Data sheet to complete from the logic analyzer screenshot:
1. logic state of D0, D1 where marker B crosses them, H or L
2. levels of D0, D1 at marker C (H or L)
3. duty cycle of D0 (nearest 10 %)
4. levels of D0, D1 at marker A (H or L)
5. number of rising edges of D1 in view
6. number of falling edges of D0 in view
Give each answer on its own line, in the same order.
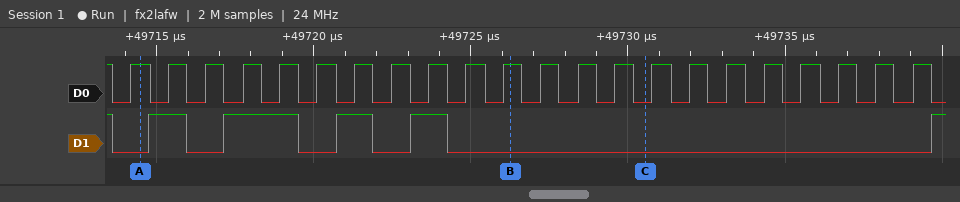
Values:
D0=H, D1=L
D0=L, D1=L
50 %
D0=H, D1=L
5
23
